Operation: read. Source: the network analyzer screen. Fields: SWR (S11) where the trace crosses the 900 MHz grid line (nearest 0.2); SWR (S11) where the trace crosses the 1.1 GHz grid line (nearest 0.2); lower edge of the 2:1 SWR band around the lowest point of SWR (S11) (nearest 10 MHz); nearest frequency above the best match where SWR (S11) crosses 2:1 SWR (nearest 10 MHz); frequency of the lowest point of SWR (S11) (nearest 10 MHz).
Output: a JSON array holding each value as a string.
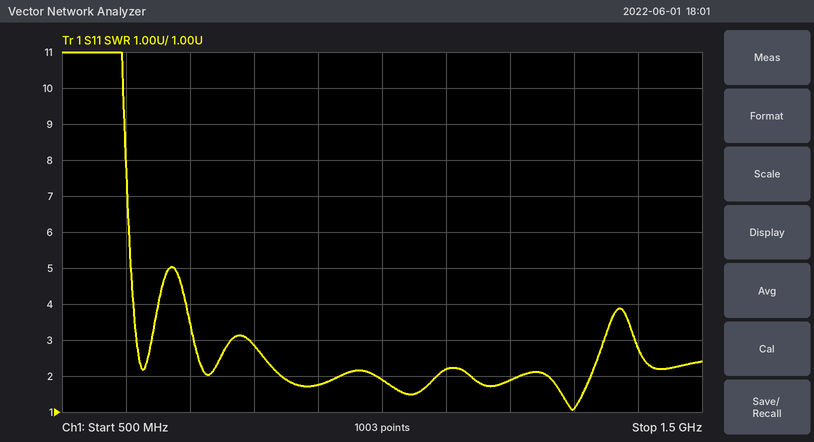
["1.8", "2.2", "1.26 GHz", "1.33 GHz", "1.30 GHz"]
